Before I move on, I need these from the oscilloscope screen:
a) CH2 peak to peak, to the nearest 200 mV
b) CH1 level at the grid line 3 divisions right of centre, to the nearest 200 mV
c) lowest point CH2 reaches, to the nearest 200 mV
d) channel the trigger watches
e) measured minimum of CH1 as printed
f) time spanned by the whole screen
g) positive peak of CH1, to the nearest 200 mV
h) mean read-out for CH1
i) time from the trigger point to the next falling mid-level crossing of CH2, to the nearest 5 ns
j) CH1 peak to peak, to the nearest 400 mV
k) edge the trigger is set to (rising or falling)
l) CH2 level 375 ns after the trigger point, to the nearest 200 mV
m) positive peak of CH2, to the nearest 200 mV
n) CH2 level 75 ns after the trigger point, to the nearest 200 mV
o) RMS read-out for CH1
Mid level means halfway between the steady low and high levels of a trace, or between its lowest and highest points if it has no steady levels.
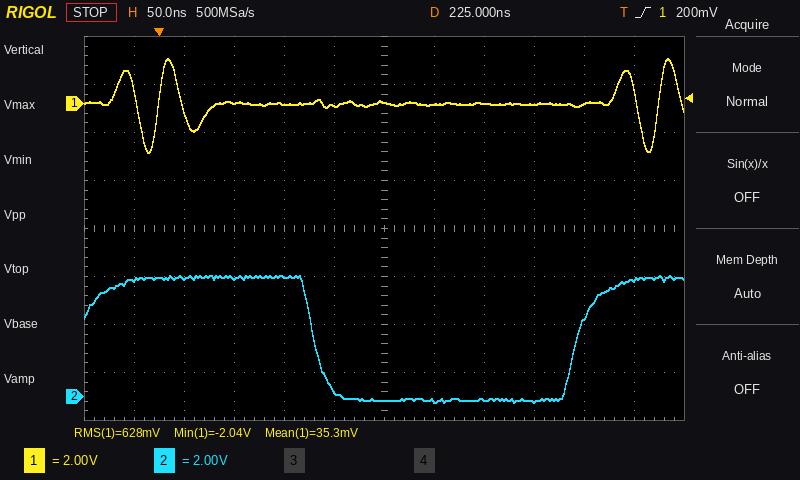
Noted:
5.2 V
0.0 V
-200 mV
CH1
-2.04 V
600 ns
1.8 V
35.3 mV
155 ns
4.0 V
rising
-200 mV
5.0 V
5.0 V
628 mV
